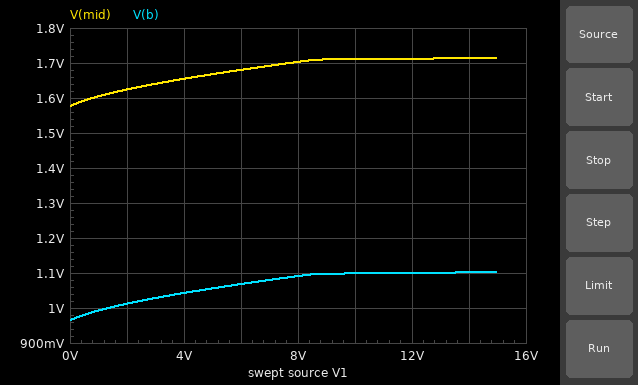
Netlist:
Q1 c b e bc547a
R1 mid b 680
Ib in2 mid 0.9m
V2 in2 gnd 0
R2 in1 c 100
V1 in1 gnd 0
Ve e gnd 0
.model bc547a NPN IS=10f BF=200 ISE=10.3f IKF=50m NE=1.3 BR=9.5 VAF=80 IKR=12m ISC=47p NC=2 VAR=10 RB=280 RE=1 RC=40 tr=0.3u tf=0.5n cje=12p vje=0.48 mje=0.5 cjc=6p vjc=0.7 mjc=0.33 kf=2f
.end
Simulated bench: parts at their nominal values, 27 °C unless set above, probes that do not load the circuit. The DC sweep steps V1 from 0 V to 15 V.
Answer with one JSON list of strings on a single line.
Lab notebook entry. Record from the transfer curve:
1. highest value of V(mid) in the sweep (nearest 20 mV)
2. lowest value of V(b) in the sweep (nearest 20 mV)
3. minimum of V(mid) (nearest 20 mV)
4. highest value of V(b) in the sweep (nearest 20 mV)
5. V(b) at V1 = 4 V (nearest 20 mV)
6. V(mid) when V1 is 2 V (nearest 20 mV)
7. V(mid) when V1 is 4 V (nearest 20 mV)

["1.72 V", "960 mV", "1.58 V", "1.10 V", "1.04 V", "1.62 V", "1.66 V"]
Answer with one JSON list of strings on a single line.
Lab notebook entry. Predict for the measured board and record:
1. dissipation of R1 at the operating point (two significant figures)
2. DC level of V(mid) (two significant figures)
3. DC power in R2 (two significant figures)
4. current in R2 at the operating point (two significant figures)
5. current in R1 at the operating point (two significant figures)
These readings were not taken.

["550 µW", "1.6 V", "130 nW", "36 µA", "900 µA"]
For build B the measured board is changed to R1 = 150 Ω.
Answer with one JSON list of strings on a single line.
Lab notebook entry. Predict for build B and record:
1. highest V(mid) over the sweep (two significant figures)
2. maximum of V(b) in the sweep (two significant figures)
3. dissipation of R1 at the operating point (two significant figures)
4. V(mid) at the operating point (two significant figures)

["1.2 V", "1.1 V", "120 µW", "1.1 V"]
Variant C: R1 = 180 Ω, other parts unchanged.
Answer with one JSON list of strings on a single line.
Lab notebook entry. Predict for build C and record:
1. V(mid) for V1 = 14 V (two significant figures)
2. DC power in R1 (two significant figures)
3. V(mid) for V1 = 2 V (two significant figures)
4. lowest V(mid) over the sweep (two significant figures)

["1.3 V", "150 µW", "1.2 V", "1.1 V"]
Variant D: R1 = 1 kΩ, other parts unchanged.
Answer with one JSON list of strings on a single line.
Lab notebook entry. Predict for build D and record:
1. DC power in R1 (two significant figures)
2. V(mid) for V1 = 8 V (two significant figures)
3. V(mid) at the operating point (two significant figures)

["810 µW", "2.0 V", "1.9 V"]
